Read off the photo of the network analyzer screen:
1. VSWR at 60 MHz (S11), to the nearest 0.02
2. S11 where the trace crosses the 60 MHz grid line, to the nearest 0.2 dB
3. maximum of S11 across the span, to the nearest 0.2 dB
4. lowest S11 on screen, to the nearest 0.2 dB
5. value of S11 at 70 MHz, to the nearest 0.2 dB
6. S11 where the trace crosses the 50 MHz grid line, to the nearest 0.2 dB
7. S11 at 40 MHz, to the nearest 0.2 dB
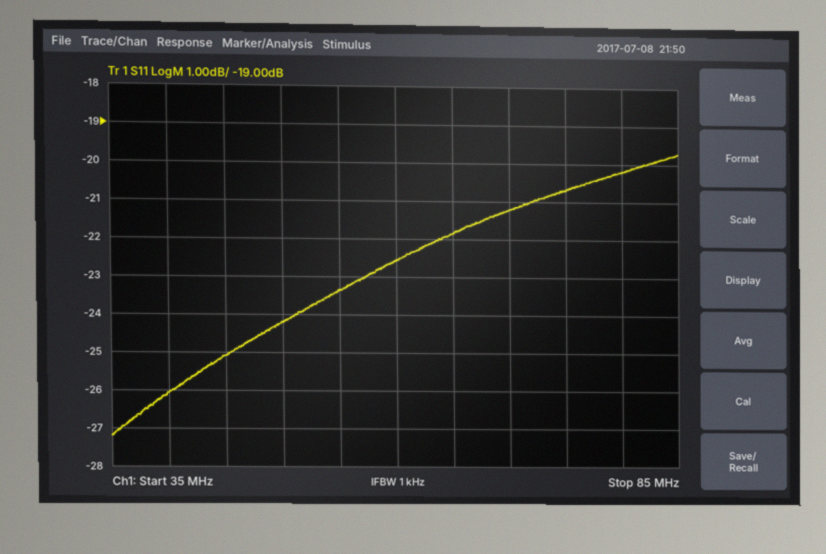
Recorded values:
1.16
-22.6 dB
-19.8 dB
-27.2 dB
-21.2 dB
-24.2 dB
-26.0 dB
